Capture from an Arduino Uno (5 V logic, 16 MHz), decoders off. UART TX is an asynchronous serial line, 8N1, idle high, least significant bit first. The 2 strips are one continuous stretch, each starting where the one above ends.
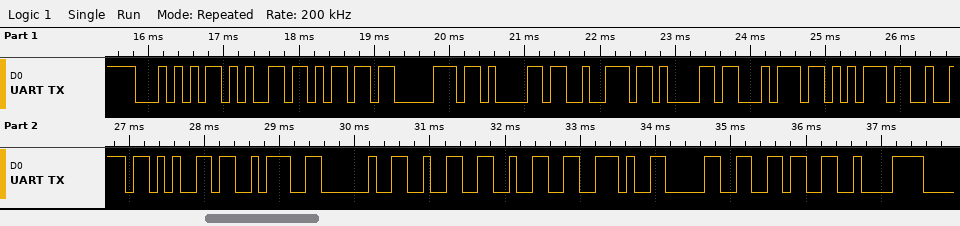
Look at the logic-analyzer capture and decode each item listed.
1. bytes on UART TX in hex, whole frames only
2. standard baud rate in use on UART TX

0x54 0x65 0x6D 0x70 0x61 0x72 0x61 0x74 0x75 0x72 0x65 0x3A 0x20 0x32 0x32 0x2E 0x30 0x36 0xC2
9600 baud
